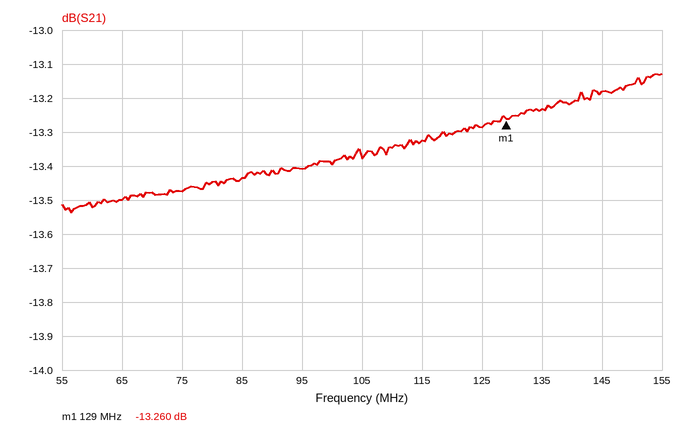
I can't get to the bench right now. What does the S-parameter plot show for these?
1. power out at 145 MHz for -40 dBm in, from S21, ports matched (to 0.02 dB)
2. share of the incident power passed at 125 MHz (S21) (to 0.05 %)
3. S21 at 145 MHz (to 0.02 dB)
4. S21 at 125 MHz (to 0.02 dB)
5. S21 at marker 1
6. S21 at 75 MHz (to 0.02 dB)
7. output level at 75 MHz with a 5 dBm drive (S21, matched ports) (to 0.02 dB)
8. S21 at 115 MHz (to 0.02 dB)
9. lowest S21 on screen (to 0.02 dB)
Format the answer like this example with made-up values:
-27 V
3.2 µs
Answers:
-53.18 dBm
4.70 %
-13.18 dB
-13.28 dB
-13.260 dB
-13.48 dB
-8.48 dBm
-13.32 dB
-13.54 dB
